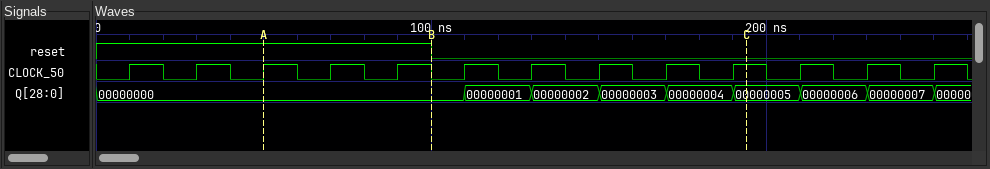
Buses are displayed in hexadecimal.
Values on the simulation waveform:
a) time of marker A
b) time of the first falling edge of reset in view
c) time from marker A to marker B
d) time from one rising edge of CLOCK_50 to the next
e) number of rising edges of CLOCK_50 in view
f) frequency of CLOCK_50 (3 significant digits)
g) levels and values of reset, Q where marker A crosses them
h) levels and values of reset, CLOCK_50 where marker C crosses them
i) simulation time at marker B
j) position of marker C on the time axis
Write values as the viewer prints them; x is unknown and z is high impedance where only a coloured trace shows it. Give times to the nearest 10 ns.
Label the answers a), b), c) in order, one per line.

a) 50 ns
b) 100 ns
c) 50 ns
d) 20 ns
e) 13
f) 50.0 MHz
g) reset=1, Q=00000000
h) reset=0, CLOCK_50=1
i) 100 ns
j) 190 ns
